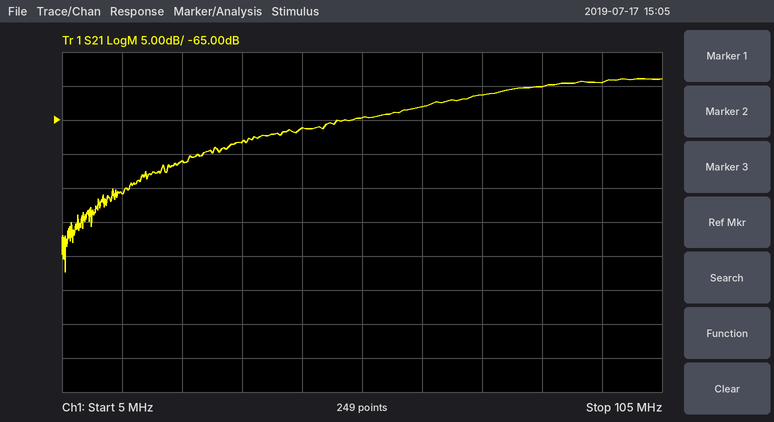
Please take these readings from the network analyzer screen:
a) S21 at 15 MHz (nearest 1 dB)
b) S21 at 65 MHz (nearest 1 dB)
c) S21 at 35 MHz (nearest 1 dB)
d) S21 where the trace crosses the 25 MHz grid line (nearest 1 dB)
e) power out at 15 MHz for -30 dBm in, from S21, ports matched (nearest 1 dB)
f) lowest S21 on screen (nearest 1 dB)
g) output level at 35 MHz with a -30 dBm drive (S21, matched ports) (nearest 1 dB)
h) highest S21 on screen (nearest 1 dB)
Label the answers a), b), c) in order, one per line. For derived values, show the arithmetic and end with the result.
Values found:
a) -76 dB
b) -63 dB
c) -68 dB
d) -71 dB
e) -30 dBm + (-76 dB) = -106 dBm
f) -87 dB
g) -30 dBm + (-68 dB) = -98 dBm
h) -59 dB
